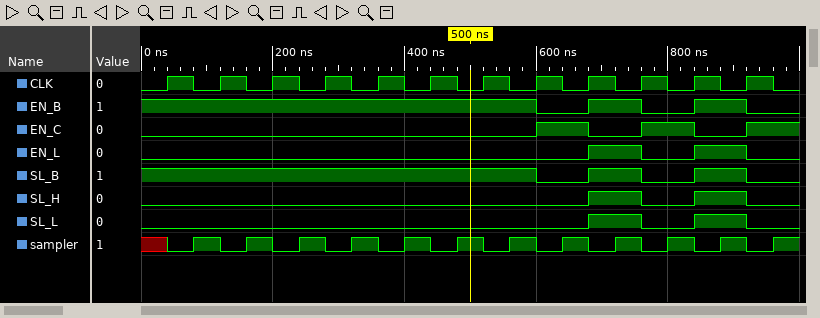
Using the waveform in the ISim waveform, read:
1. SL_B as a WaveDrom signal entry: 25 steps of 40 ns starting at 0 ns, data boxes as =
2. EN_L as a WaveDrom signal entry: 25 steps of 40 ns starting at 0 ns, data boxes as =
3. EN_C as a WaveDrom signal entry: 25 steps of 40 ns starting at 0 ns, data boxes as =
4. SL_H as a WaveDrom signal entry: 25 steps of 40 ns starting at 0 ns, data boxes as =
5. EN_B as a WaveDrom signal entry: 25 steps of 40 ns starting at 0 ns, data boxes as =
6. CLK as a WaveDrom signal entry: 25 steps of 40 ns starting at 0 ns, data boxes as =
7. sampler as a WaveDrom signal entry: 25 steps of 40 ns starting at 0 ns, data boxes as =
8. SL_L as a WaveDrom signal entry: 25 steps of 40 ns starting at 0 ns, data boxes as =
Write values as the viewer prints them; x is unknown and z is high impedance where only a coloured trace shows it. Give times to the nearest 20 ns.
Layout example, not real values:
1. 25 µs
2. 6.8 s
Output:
1. {name: 'SL_B', wave: '1..............0.1.0.1.0.'}
2. {name: 'EN_L', wave: '0................1.0.1.0.'}
3. {name: 'EN_C', wave: '0..............1.0.1.0.1.'}
4. {name: 'SL_H', wave: '0................1.0.1.0.'}
5. {name: 'EN_B', wave: '1..............0.1.0.1.0.'}
6. {name: 'CLK', wave: '0101010101010101010101010'}
7. {name: 'sampler', wave: 'x010101010101010101010101'}
8. {name: 'SL_L', wave: '0................1.0.1.0.'}
